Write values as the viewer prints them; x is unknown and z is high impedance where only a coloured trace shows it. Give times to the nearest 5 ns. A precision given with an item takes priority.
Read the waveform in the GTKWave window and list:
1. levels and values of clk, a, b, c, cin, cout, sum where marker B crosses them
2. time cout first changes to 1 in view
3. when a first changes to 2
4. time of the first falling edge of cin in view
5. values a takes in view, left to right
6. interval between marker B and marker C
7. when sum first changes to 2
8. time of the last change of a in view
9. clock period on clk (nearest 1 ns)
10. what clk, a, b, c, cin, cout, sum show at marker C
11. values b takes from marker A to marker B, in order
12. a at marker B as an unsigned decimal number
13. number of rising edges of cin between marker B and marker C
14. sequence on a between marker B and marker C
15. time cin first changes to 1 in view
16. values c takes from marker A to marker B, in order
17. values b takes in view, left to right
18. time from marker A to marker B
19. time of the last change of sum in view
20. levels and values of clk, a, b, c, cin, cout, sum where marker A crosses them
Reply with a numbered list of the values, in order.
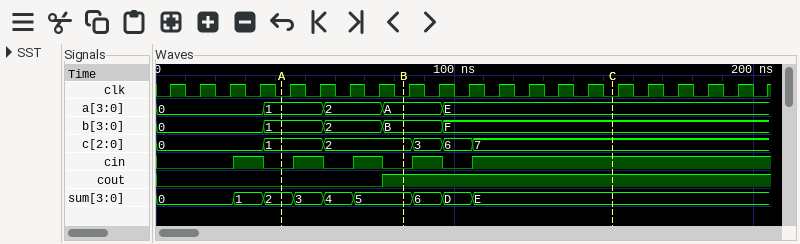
1. clk=0, a=A, b=B, c=2, cin=0, cout=1, sum=5
2. 75 ns
3. 55 ns
4. 35 ns
5. 0, 1, 2, A, E
6. 70 ns
7. 35 ns
8. 95 ns
9. 10 ns
10. clk=0, a=E, b=F, c=7, cin=1, cout=1, sum=E
11. 1, 2, B
12. 10
13. 2
14. A, E
15. 25 ns
16. 1, 2
17. 0, 1, 2, B, F
18. 40 ns
19. 105 ns
20. clk=0, a=1, b=1, c=1, cin=0, cout=0, sum=2
